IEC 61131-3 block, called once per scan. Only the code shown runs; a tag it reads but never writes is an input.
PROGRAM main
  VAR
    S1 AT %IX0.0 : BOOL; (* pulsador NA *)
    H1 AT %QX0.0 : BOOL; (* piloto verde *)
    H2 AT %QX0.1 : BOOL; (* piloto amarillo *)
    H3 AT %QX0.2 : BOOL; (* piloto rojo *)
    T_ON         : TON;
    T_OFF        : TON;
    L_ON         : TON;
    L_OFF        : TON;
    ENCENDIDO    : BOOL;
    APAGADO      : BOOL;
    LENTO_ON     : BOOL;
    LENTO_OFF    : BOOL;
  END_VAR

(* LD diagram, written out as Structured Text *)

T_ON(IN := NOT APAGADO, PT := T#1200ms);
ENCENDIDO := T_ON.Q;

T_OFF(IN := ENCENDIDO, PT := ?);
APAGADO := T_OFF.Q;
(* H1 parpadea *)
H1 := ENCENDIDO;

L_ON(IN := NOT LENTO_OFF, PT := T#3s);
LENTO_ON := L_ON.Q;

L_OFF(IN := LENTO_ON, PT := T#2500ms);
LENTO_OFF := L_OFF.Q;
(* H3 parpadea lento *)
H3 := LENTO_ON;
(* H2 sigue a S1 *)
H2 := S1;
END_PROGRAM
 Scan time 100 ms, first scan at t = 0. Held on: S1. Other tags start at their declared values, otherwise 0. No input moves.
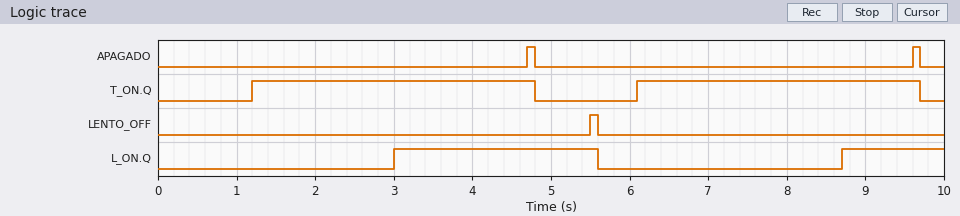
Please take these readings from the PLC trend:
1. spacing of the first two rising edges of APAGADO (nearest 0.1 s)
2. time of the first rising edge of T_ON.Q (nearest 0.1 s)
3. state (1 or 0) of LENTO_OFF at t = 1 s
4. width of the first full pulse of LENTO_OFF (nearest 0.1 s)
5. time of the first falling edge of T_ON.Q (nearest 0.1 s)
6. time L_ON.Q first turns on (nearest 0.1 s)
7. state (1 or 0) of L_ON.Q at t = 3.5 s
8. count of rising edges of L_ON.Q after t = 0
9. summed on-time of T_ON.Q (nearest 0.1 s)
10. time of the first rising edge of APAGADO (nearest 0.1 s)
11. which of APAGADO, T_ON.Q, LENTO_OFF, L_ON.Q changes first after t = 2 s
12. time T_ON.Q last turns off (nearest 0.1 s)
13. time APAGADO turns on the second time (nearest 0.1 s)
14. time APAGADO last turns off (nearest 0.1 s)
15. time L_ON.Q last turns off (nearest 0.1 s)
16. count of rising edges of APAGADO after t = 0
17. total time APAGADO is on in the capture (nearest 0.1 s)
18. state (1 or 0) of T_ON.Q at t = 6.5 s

4.9 s
1.2 s
0
0.1 s
4.8 s
3.0 s
1
2
7.2 s
4.7 s
L_ON.Q
9.7 s
9.6 s
9.7 s
5.6 s
2
0.2 s
1
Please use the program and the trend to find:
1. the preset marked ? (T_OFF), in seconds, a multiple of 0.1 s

3.5 s
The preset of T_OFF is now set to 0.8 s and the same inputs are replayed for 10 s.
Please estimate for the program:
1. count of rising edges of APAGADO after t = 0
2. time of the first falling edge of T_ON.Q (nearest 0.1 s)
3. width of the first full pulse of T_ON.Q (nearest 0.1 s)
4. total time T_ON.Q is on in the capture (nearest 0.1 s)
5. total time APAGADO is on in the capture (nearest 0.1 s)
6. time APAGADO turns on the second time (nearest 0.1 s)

4
2.1 s
0.9 s
3.6 s
0.4 s
4.2 s
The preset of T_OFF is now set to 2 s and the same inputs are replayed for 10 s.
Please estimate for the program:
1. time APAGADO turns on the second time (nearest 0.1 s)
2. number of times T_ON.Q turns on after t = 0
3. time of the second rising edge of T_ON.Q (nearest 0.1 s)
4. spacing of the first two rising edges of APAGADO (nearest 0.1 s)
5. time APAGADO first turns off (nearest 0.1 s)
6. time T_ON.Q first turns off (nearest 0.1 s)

6.6 s
3
4.6 s
3.4 s
3.3 s
3.3 s
